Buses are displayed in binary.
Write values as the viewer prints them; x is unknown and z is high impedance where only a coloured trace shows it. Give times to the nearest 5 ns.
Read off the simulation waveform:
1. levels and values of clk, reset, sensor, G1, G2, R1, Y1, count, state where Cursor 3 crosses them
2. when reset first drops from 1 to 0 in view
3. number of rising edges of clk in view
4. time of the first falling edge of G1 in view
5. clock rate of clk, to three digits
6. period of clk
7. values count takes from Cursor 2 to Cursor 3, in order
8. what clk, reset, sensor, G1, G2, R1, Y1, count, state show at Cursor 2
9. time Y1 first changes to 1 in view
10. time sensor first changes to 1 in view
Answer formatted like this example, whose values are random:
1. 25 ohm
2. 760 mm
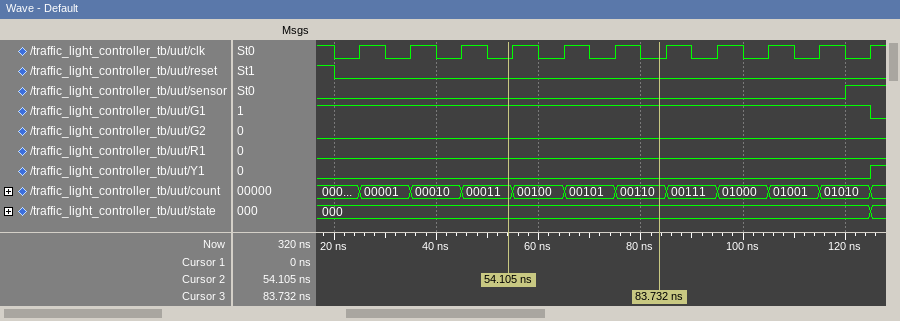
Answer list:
1. clk=0, reset=0, sensor=0, G1=1, G2=0, R1=0, Y1=0, count=00110, state=000
2. 20 ns
3. 11
4. 125 ns
5. 100 MHz
6. 10 ns
7. 00011, 00100, 00101, 00110
8. clk=0, reset=0, sensor=0, G1=1, G2=0, R1=0, Y1=0, count=00011, state=000
9. 125 ns
10. 120 ns
